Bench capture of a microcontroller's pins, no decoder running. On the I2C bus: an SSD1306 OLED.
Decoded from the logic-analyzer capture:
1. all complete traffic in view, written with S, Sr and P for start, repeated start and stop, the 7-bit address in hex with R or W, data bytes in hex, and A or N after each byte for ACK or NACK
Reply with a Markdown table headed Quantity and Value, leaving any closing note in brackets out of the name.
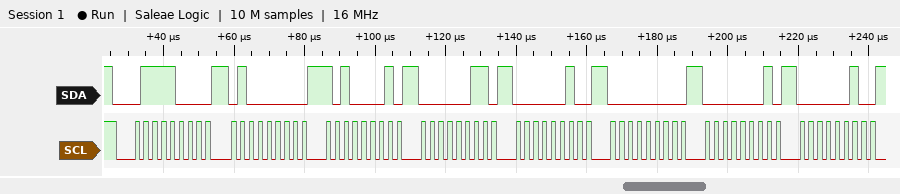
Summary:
| Quantity | Value |
|---|---|
| all complete traffic in view, written with S, Sr and P for start, repeated start and stop, the 7-bit address in hex with R or W, data bytes in hex, and A or N after each byte for ACK or NACK | S 3CW A 40 A A1 A 03 A 02 A 00 A 01 A 02 A |
